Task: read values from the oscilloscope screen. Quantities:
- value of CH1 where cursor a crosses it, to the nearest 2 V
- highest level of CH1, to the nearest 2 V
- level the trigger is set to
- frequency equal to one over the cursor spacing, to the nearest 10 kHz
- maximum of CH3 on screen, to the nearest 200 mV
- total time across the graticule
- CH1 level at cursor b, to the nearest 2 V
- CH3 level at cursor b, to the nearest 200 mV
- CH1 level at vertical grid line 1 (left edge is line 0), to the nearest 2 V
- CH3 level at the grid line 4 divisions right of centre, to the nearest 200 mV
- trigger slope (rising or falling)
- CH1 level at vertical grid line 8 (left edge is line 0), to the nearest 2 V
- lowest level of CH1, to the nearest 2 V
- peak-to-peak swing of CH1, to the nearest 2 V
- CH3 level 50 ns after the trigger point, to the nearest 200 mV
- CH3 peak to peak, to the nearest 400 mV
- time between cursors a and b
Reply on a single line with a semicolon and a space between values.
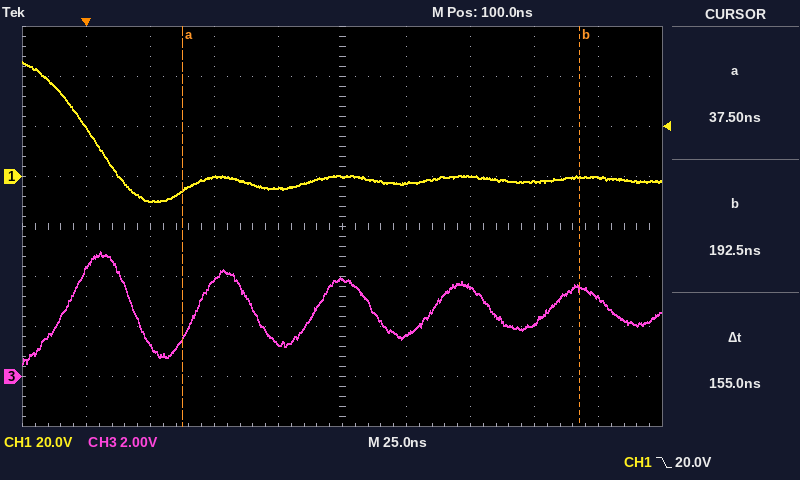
-6 V; 46 V; 20.0 V; 6.45 MHz; 5.0 V; 250 ns; 0 V; 3.6 V; 20 V; 3.2 V; falling; -2 V; -10 V; 56 V; 3.8 V; 4.4 V; 155 ns
